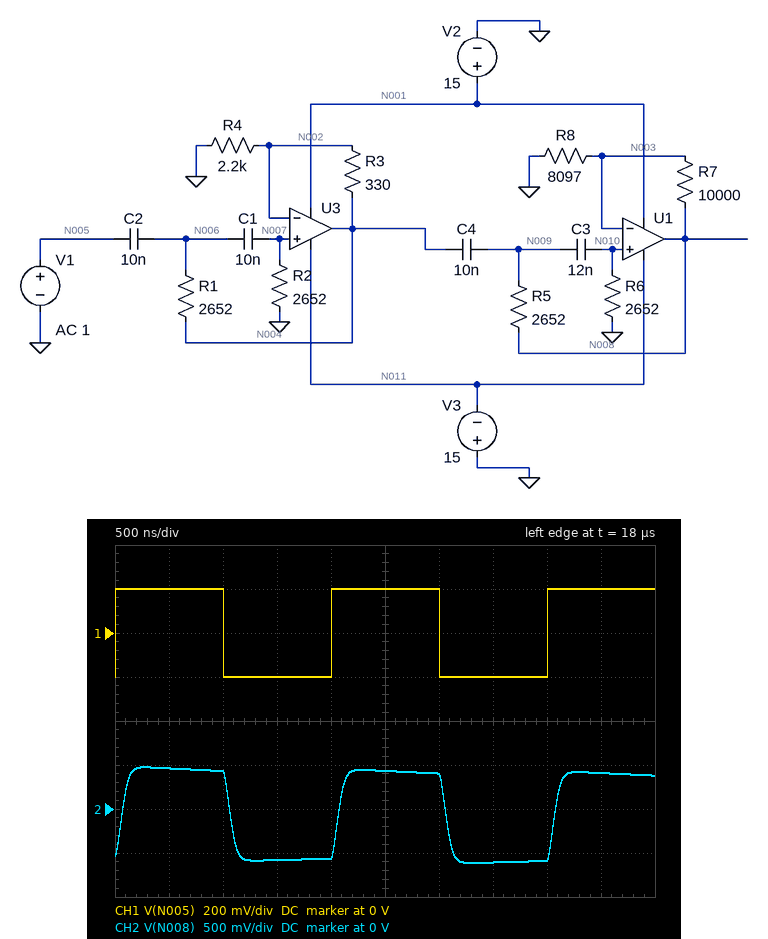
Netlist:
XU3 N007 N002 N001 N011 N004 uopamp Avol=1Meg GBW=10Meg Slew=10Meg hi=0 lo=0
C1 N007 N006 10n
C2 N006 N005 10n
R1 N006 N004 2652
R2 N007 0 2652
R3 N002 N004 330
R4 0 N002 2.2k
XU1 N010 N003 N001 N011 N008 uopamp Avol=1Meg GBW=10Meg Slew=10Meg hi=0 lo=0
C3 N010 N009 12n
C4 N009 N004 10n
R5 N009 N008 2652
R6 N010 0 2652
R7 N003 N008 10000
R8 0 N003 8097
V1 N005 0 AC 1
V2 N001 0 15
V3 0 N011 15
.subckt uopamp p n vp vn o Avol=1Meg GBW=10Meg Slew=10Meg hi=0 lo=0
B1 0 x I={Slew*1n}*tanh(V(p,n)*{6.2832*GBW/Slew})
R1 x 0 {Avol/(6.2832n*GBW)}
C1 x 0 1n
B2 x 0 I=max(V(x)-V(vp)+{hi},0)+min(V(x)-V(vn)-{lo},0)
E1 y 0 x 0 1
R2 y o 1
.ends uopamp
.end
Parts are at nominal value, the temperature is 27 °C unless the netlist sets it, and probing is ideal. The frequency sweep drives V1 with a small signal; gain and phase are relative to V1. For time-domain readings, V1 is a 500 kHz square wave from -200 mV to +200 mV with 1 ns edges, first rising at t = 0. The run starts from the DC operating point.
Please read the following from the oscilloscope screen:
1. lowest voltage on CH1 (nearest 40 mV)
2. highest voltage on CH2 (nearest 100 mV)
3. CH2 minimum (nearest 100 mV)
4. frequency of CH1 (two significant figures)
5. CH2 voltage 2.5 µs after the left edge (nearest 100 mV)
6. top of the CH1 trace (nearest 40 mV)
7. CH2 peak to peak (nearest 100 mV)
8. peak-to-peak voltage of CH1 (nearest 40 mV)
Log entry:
-200 mV
500 mV
-600 mV
500 kHz
400 mV
200 mV
1.1 V
400 mV
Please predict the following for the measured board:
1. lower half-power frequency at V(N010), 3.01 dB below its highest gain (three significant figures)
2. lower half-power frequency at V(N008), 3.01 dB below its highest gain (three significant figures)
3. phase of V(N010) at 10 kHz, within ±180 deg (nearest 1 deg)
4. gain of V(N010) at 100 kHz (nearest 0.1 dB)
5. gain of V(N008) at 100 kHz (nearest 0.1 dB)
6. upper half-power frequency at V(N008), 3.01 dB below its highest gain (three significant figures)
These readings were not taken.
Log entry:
5.33 kHz
5.33 kHz
87 deg
1.2 dB
8.2 dB
3.73 MHz
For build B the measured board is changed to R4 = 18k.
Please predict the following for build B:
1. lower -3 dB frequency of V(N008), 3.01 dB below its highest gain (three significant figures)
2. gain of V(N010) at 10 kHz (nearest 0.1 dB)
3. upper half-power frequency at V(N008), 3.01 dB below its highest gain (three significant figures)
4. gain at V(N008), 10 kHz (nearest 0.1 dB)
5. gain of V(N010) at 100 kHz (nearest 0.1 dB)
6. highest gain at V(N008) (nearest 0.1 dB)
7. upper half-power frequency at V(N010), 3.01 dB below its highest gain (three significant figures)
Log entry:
5.49 kHz
-0.4 dB
3.85 MHz
6.6 dB
0.1 dB
7.1 dB
9.88 MHz
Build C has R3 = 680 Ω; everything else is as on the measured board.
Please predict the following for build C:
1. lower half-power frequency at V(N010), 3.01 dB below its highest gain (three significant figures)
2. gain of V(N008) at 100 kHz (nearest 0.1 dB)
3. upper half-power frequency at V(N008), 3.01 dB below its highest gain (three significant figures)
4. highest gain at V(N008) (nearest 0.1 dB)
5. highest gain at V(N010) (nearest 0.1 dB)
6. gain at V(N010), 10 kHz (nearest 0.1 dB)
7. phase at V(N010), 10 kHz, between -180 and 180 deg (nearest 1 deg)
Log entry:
5.29 kHz
9.3 dB
3.14 MHz
9.9 dB
2.9 dB
2.8 dB
85 deg
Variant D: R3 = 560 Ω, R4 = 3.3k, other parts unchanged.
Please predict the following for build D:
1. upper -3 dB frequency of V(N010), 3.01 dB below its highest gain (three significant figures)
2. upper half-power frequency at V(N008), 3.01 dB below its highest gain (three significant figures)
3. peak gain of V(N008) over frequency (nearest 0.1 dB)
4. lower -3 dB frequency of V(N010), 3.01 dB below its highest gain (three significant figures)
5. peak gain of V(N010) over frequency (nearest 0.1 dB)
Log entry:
8.57 MHz
3.70 MHz
8.3 dB
5.31 kHz
1.3 dB
